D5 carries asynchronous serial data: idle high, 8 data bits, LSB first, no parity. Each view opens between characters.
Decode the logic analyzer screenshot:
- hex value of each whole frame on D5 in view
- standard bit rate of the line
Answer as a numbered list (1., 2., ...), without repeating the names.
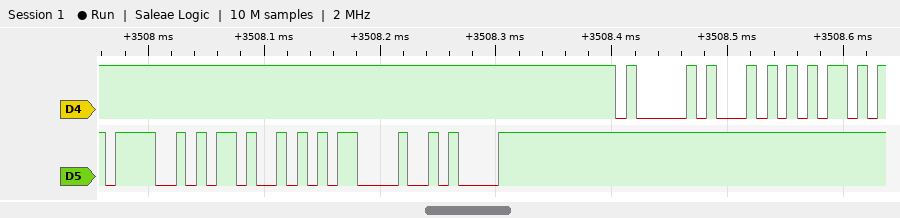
1. 4F, 4B, 0D, 0A
2. 115200 baud
